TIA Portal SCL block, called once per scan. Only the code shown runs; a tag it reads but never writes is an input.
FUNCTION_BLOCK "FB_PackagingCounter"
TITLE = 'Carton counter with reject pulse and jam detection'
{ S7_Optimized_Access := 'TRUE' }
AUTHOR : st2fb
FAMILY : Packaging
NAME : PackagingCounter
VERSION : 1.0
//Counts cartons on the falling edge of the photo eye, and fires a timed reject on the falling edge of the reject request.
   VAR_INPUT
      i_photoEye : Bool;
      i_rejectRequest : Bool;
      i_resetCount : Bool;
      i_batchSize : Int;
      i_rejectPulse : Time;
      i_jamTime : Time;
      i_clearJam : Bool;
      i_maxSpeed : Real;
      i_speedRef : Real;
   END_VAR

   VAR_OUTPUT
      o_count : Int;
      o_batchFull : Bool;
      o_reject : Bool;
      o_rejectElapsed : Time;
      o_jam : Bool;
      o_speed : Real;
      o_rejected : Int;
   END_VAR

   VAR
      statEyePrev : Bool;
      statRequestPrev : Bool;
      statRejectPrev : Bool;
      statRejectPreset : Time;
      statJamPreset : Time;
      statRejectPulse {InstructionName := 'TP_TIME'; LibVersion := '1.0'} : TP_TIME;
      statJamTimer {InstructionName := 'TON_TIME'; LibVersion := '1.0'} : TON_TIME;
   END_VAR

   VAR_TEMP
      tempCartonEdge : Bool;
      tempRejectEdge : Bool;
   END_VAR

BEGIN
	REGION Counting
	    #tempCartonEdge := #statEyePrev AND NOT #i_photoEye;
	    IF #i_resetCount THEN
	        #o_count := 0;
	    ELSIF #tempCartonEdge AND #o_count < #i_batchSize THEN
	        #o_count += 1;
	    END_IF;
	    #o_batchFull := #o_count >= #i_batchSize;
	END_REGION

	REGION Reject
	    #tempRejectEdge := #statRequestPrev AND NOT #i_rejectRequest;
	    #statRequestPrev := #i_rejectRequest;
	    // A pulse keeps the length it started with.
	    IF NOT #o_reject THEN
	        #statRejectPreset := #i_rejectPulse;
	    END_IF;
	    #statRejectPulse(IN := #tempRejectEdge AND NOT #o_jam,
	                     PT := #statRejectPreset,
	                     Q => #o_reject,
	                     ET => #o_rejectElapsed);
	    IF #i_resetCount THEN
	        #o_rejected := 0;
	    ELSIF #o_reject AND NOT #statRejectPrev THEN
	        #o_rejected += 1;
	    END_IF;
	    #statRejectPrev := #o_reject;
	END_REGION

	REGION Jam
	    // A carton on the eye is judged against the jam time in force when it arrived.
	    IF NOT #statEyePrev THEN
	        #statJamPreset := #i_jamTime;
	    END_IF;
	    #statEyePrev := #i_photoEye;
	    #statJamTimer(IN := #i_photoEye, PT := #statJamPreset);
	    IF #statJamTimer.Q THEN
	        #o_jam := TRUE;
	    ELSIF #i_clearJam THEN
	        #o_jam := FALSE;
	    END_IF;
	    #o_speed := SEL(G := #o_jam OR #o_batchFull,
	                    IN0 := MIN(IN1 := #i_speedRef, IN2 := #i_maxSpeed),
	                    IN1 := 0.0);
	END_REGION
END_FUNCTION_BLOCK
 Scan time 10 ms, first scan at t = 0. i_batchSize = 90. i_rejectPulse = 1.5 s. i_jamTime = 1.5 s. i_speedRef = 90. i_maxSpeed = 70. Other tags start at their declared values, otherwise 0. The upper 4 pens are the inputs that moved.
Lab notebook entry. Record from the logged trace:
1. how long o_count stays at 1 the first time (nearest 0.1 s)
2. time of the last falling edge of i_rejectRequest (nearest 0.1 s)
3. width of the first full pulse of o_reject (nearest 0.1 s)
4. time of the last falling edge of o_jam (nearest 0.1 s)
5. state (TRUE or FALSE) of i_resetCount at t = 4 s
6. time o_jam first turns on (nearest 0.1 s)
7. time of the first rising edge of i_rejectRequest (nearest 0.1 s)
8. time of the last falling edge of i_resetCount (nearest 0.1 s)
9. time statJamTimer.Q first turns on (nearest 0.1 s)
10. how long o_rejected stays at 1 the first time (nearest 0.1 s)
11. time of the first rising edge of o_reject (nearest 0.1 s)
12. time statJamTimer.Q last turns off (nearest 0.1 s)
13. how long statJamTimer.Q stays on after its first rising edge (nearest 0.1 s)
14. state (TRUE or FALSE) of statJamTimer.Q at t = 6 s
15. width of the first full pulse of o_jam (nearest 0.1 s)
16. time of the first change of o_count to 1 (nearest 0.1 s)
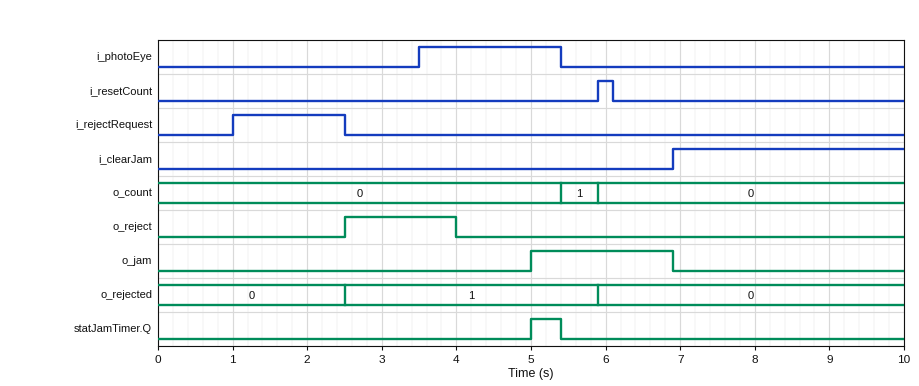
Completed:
0.5 s
2.5 s
1.5 s
6.9 s
FALSE
5.0 s
1.0 s
6.1 s
5.0 s
3.4 s
2.5 s
5.4 s
0.4 s
FALSE
1.9 s
5.4 s
